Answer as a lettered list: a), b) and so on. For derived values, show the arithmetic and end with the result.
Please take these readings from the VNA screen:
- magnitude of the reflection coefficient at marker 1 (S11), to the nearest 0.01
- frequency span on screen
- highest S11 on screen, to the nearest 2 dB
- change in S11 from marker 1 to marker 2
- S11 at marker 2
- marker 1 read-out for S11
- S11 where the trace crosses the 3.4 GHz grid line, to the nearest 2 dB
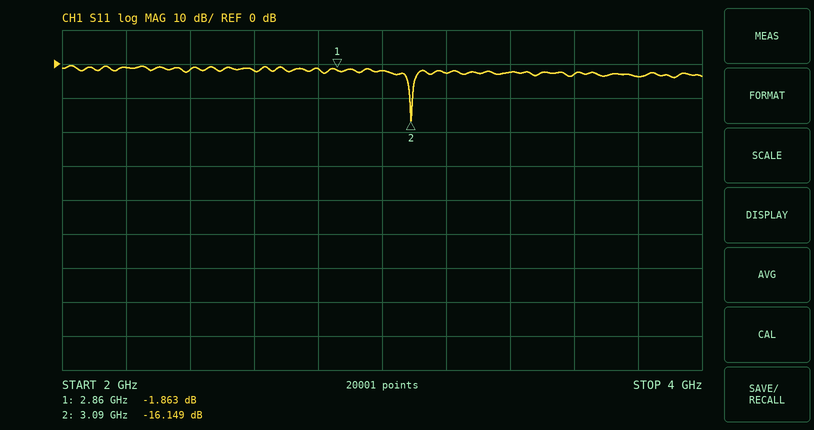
a) 10^(-1.863/20) ≈ 0.81
b) 2 GHz
c) 0 dB
d) -16.149 − (-1.863) = -14.286 dB
e) -16.149 dB
f) -1.863 dB
g) -2 dB
